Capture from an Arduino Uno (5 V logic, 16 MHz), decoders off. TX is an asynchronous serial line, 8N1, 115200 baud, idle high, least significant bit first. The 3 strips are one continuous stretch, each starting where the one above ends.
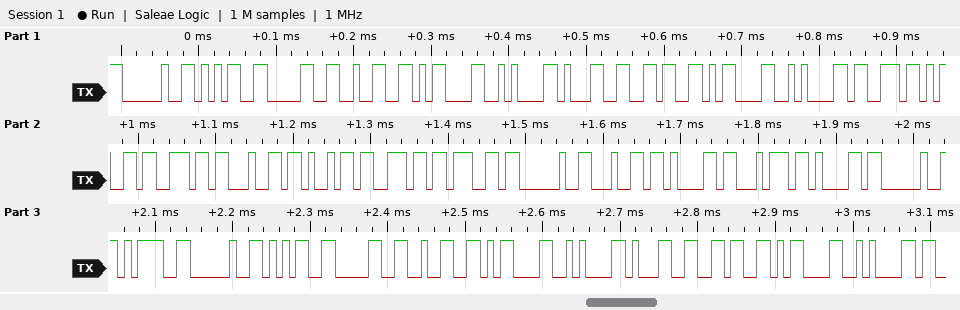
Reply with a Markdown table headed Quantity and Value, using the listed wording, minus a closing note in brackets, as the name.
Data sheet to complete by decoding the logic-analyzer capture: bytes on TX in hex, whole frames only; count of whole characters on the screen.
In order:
| Quantity | Value |
|---|---|
| bytes on TX in hex, whole frames only | 20 35 30 32 0D 0A 31 36 0D 0A 73 65 6E 64 69 6E 67 20 64 61 74 61 20 3D 20 35 30 32 0D 0A 31 36 0D 0A |
| count of whole characters on the screen | 34 |
